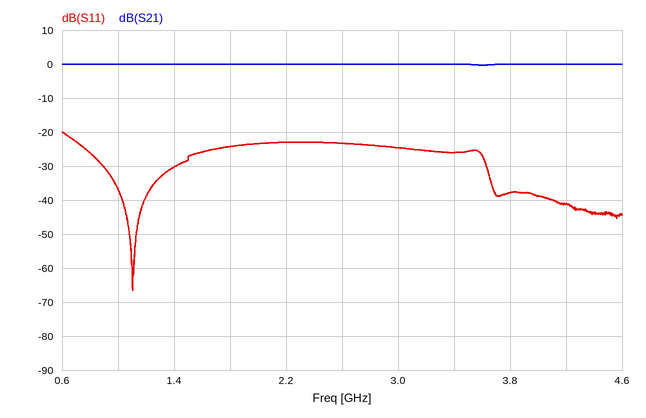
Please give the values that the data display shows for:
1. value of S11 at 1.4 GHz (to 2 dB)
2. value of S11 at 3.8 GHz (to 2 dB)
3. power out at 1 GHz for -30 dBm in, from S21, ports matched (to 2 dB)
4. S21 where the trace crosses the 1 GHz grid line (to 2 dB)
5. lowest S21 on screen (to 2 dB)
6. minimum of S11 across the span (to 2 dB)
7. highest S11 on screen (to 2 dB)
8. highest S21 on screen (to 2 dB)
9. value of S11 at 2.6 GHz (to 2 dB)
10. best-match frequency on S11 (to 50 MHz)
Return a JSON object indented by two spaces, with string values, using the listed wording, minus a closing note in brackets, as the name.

{
  "value of S11 at 1.4 GHz": "-30 dB",
  "value of S11 at 3.8 GHz": "-38 dB",
  "power out at 1 GHz for -30 dBm in, from S21, ports matched": "-30 dBm",
  "S21 where the trace crosses the 1 GHz grid line": "0 dB",
  "lowest S21 on screen": "0 dB",
  "minimum of S11 across the span": "-66 dB",
  "highest S11 on screen": "-20 dB",
  "highest S21 on screen": "0 dB",
  "value of S11 at 2.6 GHz": "-24 dB",
  "best-match frequency on S11": "1.10 GHz"
}
